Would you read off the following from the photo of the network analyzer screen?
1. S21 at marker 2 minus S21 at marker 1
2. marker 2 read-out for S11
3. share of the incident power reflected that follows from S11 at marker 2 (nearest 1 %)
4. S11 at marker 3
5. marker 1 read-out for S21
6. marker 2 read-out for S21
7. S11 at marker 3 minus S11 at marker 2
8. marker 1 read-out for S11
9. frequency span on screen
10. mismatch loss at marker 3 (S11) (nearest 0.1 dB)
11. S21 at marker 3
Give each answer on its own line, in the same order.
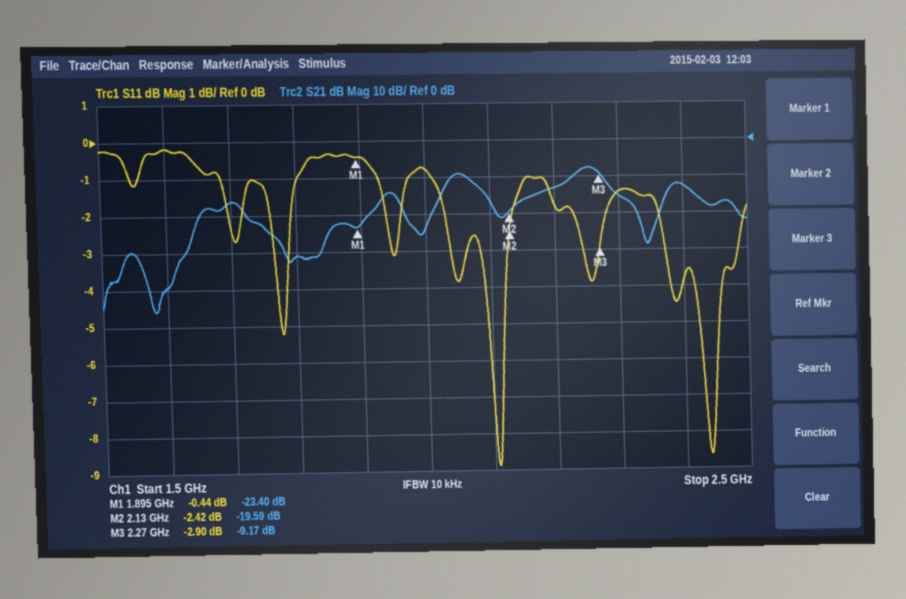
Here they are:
3.81 dB
-2.42 dB
57 %
-2.90 dB
-23.40 dB
-19.59 dB
-0.48 dB
-0.44 dB
1 GHz
3.1 dB
-9.17 dB
